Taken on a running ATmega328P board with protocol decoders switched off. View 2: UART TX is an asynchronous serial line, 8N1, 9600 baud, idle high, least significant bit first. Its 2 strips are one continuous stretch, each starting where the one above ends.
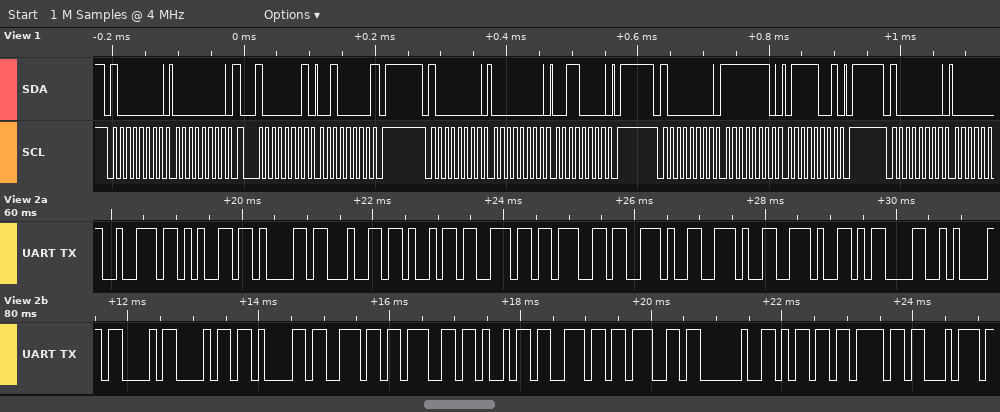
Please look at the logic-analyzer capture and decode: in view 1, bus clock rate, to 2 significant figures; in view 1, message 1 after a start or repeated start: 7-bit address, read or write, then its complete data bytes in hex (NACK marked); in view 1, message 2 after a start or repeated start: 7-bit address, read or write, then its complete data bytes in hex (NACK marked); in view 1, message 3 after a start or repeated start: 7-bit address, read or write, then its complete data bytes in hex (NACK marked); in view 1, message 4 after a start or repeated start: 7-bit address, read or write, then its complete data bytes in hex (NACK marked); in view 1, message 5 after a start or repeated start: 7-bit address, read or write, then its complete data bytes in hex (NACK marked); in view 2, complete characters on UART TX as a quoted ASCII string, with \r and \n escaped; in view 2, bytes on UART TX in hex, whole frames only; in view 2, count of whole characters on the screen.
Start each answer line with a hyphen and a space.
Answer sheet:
- 100 kHz
- 0x40 write: 00
- 0x40 read: 20 NACK
- 0x40 write: 00 30
- 0x40 write: FE 79
- 0x40 write
- "reading...\r\nChanging mot"
- 72 65 61 64 69 6E 67 2E 2E 2E 0D 0A 43 68 61 6E 67 69 6E 67 20 6D 6F 74
- 24
